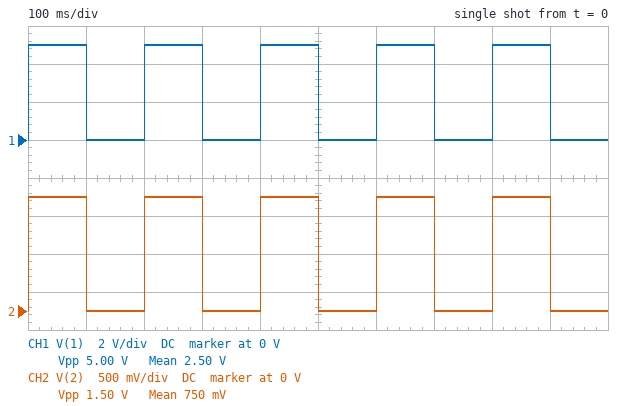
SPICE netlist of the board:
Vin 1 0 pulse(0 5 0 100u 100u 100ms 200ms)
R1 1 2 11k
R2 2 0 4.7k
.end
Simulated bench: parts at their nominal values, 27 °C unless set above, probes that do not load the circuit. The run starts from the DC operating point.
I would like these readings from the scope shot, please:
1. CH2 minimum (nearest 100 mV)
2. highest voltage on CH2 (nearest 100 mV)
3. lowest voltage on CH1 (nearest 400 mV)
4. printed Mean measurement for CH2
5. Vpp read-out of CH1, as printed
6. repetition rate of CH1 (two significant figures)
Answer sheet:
0 V
1.5 V
0 V
750 mV
5.00 V
5.0 Hz
